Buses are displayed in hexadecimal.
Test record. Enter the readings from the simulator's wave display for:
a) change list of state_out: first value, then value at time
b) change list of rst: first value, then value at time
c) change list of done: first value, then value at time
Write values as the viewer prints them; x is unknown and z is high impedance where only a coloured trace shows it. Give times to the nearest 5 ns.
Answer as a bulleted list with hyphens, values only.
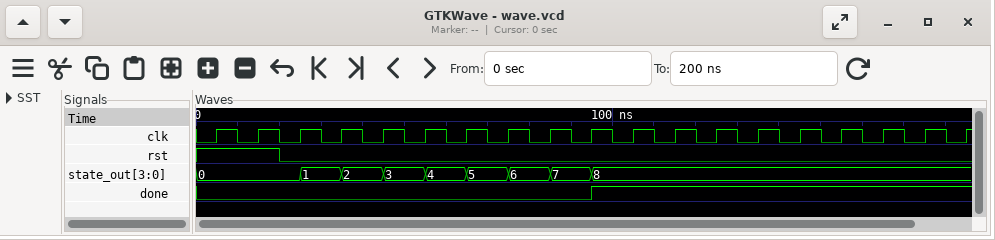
- 0, 1 at 25 ns, 2 at 35 ns, 3 at 45 ns, 4 at 55 ns, 5 at 65 ns, 6 at 75 ns, 7 at 85 ns, 8 at 95 ns
- 1, 0 at 20 ns
- 0, 1 at 95 ns
